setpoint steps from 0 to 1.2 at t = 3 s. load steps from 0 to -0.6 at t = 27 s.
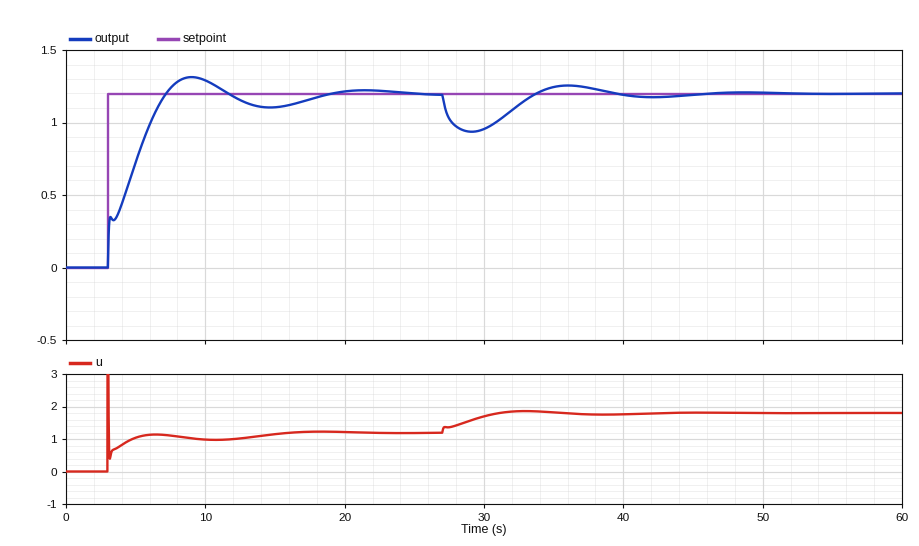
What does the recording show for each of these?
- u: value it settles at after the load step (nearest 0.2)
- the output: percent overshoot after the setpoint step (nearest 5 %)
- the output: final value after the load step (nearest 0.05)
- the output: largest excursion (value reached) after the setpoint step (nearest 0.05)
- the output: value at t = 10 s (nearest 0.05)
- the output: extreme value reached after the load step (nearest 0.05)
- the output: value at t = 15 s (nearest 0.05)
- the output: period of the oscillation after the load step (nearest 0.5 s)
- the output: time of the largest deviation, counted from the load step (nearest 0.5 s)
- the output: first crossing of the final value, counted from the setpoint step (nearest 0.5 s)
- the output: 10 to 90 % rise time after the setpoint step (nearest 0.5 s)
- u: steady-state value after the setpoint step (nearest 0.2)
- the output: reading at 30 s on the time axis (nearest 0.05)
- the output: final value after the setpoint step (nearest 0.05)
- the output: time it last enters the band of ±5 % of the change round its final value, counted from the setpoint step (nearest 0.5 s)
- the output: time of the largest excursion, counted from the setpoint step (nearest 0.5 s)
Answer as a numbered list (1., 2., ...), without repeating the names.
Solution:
1. 1.8
2. 10 %
3. 1.20
4. 1.30
5. 1.30
6. 0.95
7. 1.10
8. 13.0 s
9. 2.0 s
10. 4.0 s
11. 3.5 s
12. 1.2
13. 0.95
14. 1.20
15. 14.0 s
16. 6.0 s
